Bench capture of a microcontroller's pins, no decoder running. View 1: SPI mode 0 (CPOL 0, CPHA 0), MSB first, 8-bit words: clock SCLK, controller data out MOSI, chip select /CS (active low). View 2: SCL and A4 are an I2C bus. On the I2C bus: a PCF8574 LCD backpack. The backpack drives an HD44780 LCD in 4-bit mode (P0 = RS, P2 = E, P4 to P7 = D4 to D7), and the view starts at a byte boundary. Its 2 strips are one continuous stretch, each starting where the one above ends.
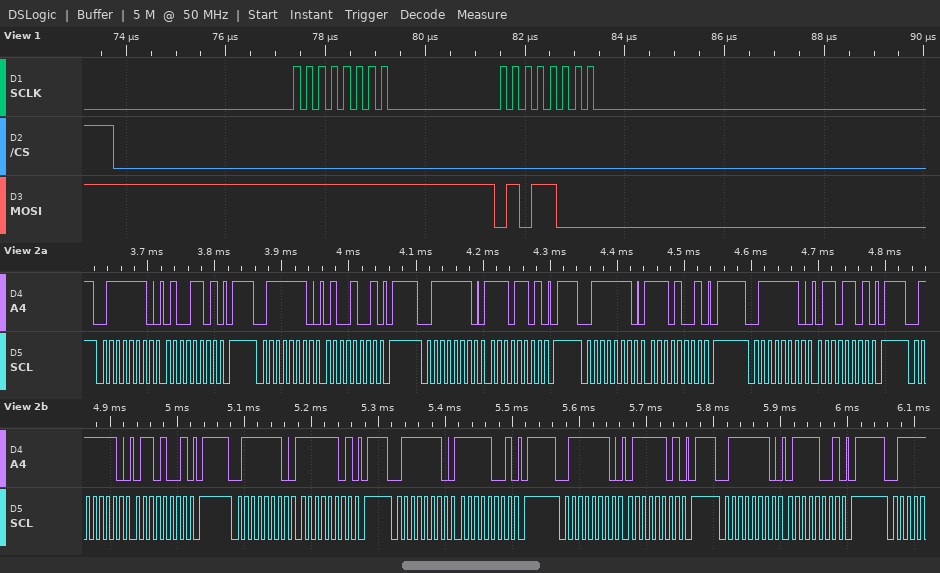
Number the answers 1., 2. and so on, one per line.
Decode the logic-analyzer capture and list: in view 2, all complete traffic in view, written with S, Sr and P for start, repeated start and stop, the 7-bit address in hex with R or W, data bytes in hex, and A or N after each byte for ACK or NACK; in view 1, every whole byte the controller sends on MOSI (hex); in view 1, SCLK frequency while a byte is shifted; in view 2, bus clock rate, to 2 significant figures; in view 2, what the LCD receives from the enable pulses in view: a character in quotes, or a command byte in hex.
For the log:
1. S 3FW A 4D A P S 3FW A 49 A P S 3FW A ED A P S 3FW A E9 A P S 3FW A 6D A P S 3FW A 69 A P S 3FW A FD A P S 3FW A F9 A P S 3FW A 7D A P S 3FW A 79 A P
2. FF 58
3. 4 MHz
4. 100 kHz
5. 'N' 'o'
